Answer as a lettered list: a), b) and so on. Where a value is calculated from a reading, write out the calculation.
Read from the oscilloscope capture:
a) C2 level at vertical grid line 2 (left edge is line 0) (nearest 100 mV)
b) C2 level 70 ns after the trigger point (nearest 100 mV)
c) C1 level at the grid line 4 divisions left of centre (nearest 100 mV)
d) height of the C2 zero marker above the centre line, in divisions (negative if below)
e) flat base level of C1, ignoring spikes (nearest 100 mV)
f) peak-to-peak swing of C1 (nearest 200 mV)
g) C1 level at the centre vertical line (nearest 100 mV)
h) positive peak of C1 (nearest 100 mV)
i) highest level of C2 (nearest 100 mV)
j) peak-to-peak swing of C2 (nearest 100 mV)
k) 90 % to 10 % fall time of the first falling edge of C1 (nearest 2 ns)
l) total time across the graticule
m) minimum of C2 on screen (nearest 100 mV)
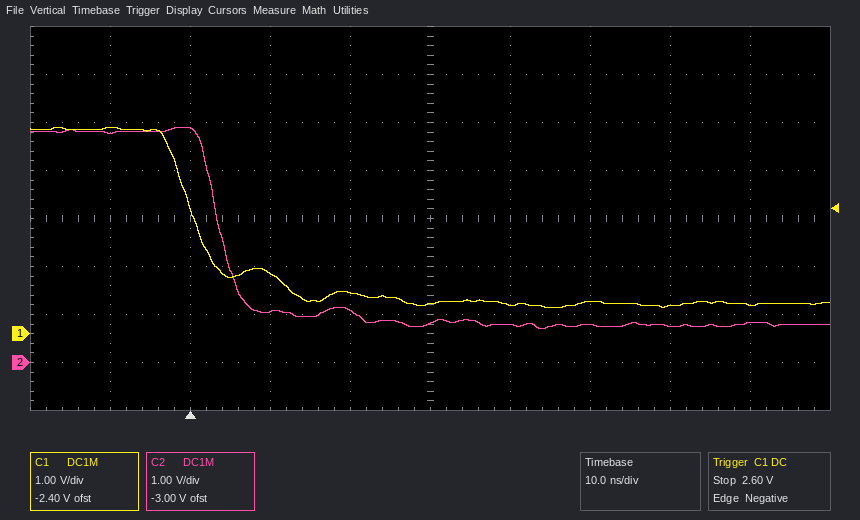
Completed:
a) 4.9 V
b) 800 mV
c) 4.3 V
d) -3.0 div
e) 600 mV
f) 3.8 V
g) 600 mV
h) 4.3 V
i) 4.9 V
j) 4.9 V − (700 mV) = 4.2 V
k) 14 ns
l) 100 ns
m) 700 mV
